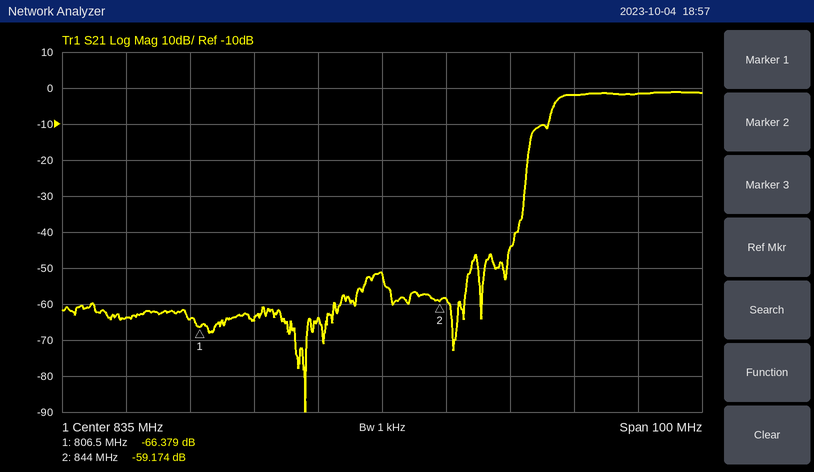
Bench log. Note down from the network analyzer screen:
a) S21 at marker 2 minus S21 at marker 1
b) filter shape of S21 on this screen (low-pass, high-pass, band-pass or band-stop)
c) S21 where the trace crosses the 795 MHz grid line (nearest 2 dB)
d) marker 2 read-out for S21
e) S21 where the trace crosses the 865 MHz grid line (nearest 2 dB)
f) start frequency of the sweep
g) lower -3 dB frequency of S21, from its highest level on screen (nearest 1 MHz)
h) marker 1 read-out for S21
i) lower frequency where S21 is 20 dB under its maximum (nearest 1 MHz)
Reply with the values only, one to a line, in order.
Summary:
7.205 dB
high-pass
-64 dB
-59.174 dB
-2 dB
785 MHz
862 MHz
-66.379 dB
858 MHz
